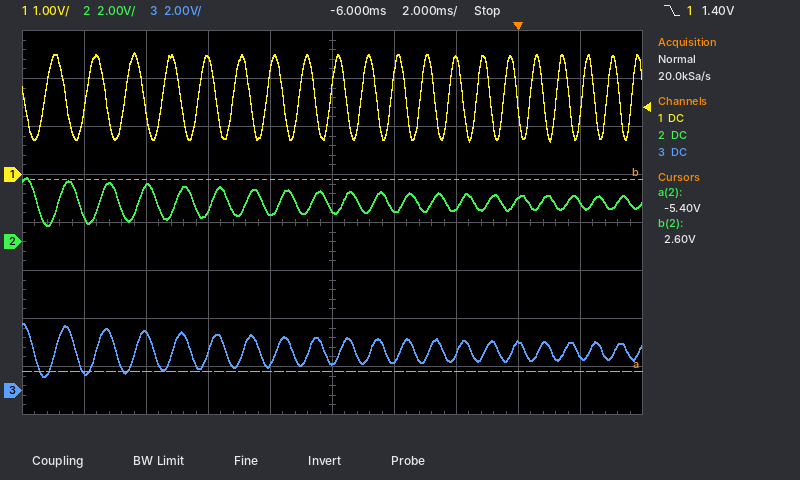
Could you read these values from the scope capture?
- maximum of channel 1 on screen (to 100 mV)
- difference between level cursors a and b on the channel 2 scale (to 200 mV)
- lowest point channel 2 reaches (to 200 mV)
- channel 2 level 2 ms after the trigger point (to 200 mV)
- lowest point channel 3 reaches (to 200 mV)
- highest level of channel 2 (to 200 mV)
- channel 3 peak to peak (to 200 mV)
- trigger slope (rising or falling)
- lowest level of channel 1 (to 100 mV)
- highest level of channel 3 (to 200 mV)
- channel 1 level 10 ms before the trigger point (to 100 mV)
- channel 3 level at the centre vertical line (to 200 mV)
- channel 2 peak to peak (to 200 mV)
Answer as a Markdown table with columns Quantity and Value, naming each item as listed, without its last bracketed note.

| Quantity | Value |
|---|---|
| maximum of channel 1 on screen | 2.5 V |
| difference between level cursors a and b on the channel 2 scale | 8.0 V |
| lowest point channel 2 reaches | 600 mV |
| channel 2 level 2 ms after the trigger point | 1.6 V |
| lowest point channel 3 reaches | 600 mV |
| highest level of channel 2 | 2.6 V |
| channel 3 peak to peak | 2.2 V |
| trigger slope | falling |
| lowest level of channel 1 | 700 mV |
| highest level of channel 3 | 2.8 V |
| channel 1 level 10 ms before the trigger point | 2.4 V |
| channel 3 level at the centre vertical line | 1.2 V |
| channel 2 peak to peak | 2.0 V |
